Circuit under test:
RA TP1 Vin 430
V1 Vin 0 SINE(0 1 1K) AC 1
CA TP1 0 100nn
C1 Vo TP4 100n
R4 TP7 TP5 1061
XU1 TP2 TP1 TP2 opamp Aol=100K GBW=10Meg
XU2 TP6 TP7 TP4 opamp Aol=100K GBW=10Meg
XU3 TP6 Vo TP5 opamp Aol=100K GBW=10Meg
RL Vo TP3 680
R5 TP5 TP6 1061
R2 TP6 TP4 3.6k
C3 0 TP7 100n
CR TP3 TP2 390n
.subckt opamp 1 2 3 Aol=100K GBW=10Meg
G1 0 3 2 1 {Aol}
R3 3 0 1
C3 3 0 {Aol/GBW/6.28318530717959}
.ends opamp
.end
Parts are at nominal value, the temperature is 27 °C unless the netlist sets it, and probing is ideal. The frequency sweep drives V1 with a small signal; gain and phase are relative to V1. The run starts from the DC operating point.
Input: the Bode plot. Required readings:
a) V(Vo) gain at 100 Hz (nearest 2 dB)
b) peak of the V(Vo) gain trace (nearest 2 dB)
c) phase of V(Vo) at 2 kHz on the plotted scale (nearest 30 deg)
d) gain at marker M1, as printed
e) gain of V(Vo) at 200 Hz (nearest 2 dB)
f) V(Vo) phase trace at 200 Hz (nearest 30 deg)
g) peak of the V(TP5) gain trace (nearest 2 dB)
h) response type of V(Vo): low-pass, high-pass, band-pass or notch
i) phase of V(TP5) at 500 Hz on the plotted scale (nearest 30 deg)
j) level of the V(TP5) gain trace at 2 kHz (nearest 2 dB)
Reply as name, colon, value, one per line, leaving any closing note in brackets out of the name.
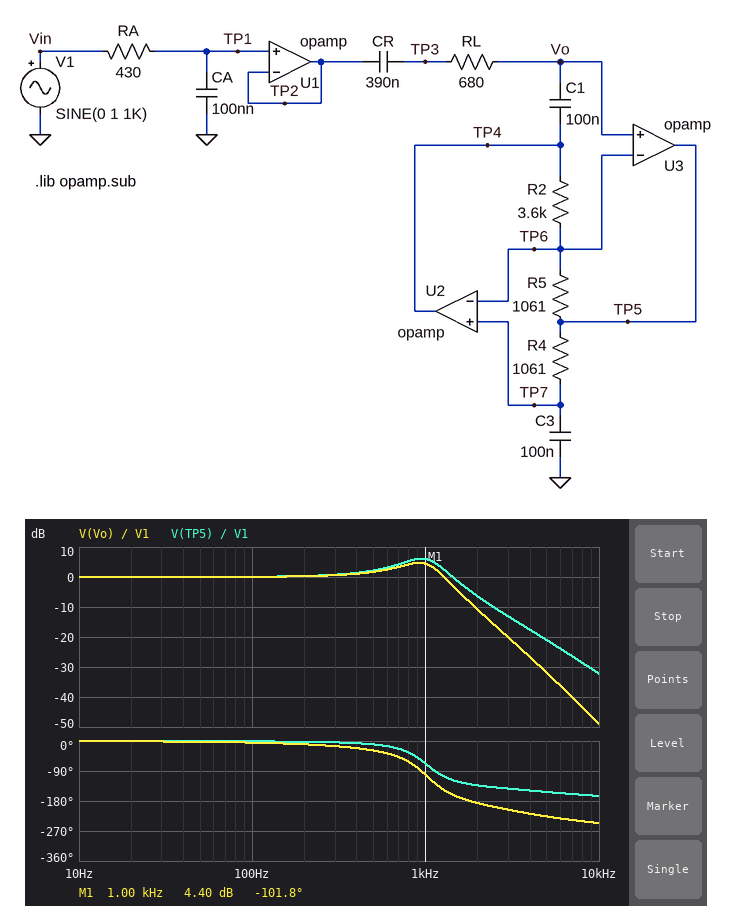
V(Vo) gain at 100 Hz: 0 dB
peak of the V(Vo) gain trace: 4 dB
phase of V(Vo) at 2 kHz on the plotted scale: -180 deg
gain at marker M1, as printed: 4.40 dB
gain of V(Vo) at 200 Hz: 0 dB
V(Vo) phase trace at 200 Hz: 0 deg
peak of the V(TP5) gain trace: 6 dB
response type of V(Vo): low-pass, high-pass, band-pass or notch: low-pass
phase of V(TP5) at 500 Hz on the plotted scale: 0 deg
level of the V(TP5) gain trace at 2 kHz: -6 dB
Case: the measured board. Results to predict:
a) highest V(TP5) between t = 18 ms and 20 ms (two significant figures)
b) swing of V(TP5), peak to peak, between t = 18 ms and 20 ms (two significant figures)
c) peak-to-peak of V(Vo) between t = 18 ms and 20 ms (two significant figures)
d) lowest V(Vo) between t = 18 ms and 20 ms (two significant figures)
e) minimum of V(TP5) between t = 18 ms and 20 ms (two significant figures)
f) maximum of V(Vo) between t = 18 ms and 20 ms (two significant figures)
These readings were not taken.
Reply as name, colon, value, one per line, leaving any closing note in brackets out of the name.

highest V(TP5) between t = 18 ms and 20 ms: 2.0 V
swing of V(TP5), peak to peak, between t = 18 ms and 20 ms: 4.0 V
peak-to-peak of V(Vo) between t = 18 ms and 20 ms: 3.3 V
lowest V(Vo) between t = 18 ms and 20 ms: -1.7 V
minimum of V(TP5) between t = 18 ms and 20 ms: -2.0 V
maximum of V(Vo) between t = 18 ms and 20 ms: 1.7 V
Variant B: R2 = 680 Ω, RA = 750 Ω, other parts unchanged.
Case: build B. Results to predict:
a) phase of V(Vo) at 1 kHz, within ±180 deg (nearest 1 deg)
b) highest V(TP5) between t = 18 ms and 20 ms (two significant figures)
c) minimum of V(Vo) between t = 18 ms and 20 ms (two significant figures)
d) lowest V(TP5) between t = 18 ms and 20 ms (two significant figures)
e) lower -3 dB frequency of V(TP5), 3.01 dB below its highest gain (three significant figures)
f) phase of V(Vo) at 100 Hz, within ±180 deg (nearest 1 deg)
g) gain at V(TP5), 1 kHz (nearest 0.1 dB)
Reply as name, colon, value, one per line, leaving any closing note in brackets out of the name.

phase of V(Vo) at 1 kHz, within ±180 deg: -33 deg
highest V(TP5) between t = 18 ms and 20 ms: 1.3 V
minimum of V(Vo) between t = 18 ms and 20 ms: -1.1 V
lowest V(TP5) between t = 18 ms and 20 ms: -1.3 V
lower -3 dB frequency of V(TP5), 3.01 dB below its highest gain: 1.99 kHz
phase of V(Vo) at 100 Hz, within ±180 deg: -3 deg
gain at V(TP5), 1 kHz: 2.4 dB
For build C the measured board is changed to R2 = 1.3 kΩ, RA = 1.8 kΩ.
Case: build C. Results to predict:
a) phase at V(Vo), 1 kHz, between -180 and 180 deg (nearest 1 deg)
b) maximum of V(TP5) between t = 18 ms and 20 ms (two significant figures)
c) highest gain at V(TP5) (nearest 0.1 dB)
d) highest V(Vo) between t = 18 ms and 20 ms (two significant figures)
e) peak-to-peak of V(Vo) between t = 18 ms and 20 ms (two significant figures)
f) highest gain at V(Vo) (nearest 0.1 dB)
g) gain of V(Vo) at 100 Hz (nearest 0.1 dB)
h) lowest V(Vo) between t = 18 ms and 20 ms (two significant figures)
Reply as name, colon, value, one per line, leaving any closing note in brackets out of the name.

phase at V(Vo), 1 kHz, between -180 and 180 deg: -66 deg
maximum of V(TP5) between t = 18 ms and 20 ms: 1.2 V
highest gain at V(TP5): 6.1 dB
highest V(Vo) between t = 18 ms and 20 ms: 970 mV
peak-to-peak of V(Vo) between t = 18 ms and 20 ms: 1.9 V
highest gain at V(Vo): 2.8 dB
gain of V(Vo) at 100 Hz: 0 dB
lowest V(Vo) between t = 18 ms and 20 ms: -970 mV
